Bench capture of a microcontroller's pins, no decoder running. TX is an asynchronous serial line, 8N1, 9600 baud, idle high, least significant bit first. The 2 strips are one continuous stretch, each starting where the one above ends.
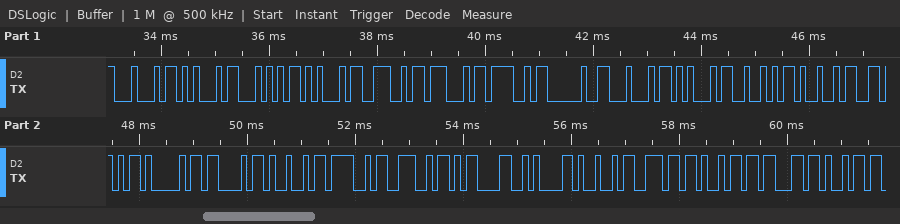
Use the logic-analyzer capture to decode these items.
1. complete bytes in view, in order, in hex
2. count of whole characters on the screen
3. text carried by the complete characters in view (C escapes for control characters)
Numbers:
0x44 0x45 0x54 0x45 0x4E 0x47 0x4F 0x20 0x44 0x45 0x52 0x49 0x56 0x41 0x43 0x49 0x4F 0x4E 0x0D 0x0A 0x49 0x6E 0x69 0x63 0x69
25
"DETENGO DERIVACION\r\nInici"
